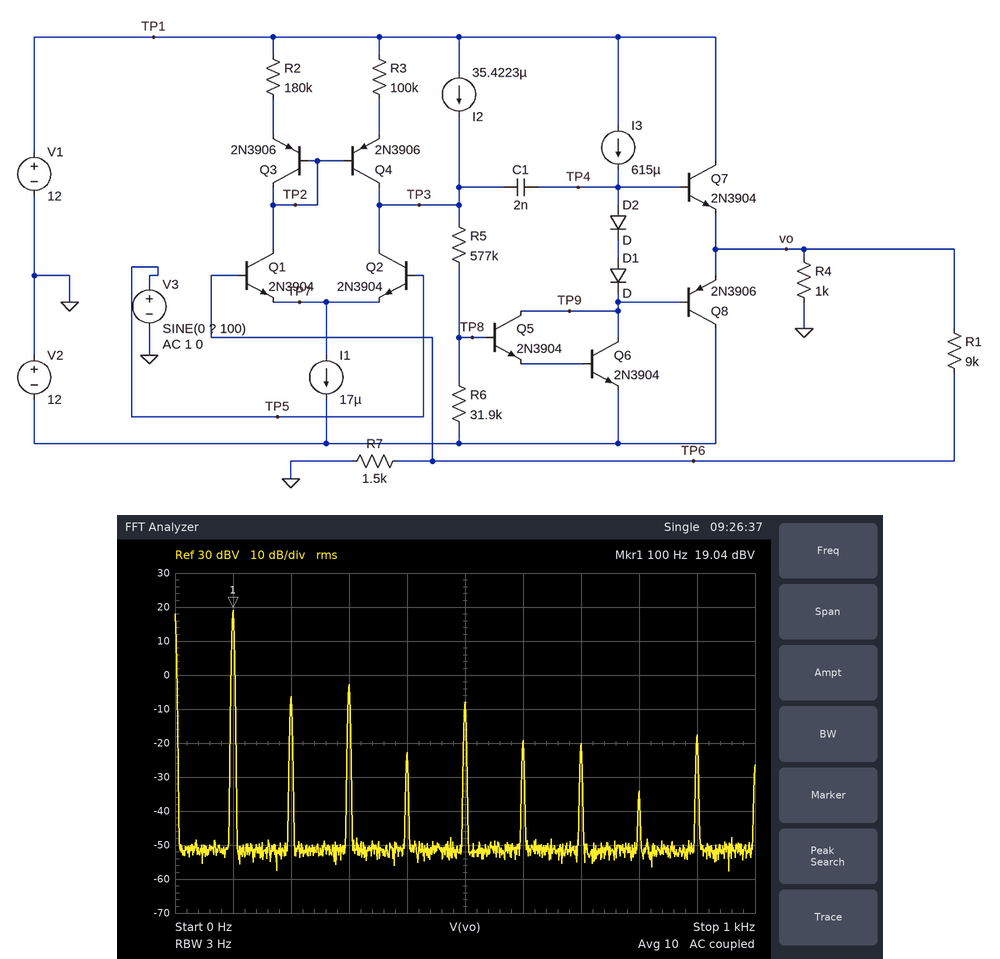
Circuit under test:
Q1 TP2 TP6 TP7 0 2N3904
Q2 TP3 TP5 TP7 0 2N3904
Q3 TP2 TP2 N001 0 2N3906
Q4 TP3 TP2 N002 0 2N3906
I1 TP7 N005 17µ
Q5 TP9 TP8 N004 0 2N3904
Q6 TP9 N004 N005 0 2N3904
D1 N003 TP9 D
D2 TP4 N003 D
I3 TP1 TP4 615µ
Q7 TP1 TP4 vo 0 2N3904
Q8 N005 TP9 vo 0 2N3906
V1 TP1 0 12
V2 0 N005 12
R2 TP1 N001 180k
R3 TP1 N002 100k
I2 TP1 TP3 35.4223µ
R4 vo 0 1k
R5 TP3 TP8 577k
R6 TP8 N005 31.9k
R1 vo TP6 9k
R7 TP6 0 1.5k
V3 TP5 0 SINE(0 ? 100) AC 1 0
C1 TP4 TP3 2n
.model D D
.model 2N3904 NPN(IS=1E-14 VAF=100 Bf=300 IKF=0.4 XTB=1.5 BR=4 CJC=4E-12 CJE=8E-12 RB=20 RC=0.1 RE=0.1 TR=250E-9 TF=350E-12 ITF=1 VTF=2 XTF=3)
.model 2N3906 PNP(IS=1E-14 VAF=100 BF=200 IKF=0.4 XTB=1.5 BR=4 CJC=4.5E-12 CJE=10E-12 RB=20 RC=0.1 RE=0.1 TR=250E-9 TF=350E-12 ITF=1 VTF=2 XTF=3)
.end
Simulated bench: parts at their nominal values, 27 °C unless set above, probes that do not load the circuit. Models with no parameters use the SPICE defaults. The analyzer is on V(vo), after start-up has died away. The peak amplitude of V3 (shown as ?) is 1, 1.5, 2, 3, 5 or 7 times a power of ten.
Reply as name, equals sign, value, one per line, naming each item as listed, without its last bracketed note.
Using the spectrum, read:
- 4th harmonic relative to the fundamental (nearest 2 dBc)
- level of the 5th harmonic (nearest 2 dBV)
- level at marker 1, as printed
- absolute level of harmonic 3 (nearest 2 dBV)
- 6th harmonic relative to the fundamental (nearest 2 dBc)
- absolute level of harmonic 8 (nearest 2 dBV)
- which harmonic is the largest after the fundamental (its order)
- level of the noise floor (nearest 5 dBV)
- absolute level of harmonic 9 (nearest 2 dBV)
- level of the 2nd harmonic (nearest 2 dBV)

4th harmonic relative to the fundamental = -42 dBc
level of the 5th harmonic = -8 dBV
level at marker 1, as printed = 19.04 dBV
absolute level of harmonic 3 = -2 dBV
6th harmonic relative to the fundamental = -38 dBc
absolute level of harmonic 8 = -34 dBV
which harmonic is the largest after the fundamental = 3
level of the noise floor = -50 dBV
absolute level of harmonic 9 = -18 dBV
level of the 2nd harmonic = -6 dBV
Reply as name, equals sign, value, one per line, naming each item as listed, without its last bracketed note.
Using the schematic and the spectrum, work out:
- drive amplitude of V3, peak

drive amplitude of V3, peak = 2 V
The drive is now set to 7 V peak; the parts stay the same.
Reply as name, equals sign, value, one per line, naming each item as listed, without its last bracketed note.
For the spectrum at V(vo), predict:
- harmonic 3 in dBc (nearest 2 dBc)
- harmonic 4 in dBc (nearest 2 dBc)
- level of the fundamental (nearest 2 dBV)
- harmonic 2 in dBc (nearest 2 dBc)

harmonic 3 in dBc = -20 dBc
harmonic 4 in dBc = -32 dBc
level of the fundamental = 20 dBV
harmonic 2 in dBc = -30 dBc
